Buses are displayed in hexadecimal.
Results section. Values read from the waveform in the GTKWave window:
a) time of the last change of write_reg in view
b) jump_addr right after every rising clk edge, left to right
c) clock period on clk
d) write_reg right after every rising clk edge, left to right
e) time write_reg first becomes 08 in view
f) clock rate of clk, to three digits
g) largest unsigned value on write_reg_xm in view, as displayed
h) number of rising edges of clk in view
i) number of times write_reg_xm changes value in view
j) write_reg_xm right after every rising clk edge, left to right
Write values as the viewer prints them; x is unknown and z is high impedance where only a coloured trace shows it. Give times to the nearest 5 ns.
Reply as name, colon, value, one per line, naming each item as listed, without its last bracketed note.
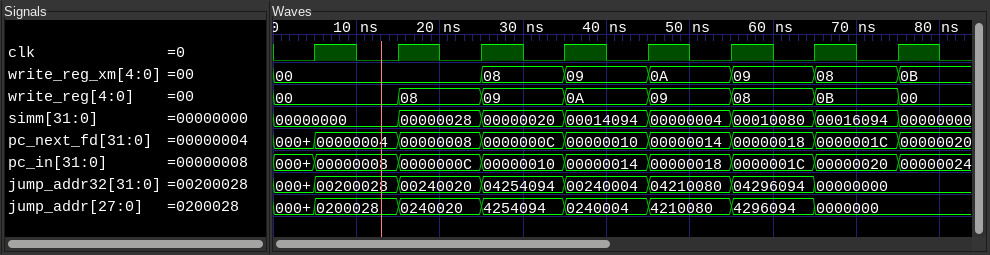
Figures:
time of the last change of write_reg in view: 75 ns
jump_addr right after every rising clk edge, left to right: 0200028, 0240020, 4254094, 0240004, 4210080, 4296094, 0000000, 0000000
clock period on clk: 10 ns
write_reg right after every rising clk edge, left to right: 00, 08, 09, 0A, 09, 08, 0B, 00
time write_reg first becomes 08 in view: 15 ns
clock rate of clk, to three digits: 100 MHz
largest unsigned value on write_reg_xm in view, as displayed: 0B
number of rising edges of clk in view: 8
number of times write_reg_xm changes value in view: 6
write_reg_xm right after every rising clk edge, left to right: 00, 00, 08, 09, 0A, 09, 08, 0B
